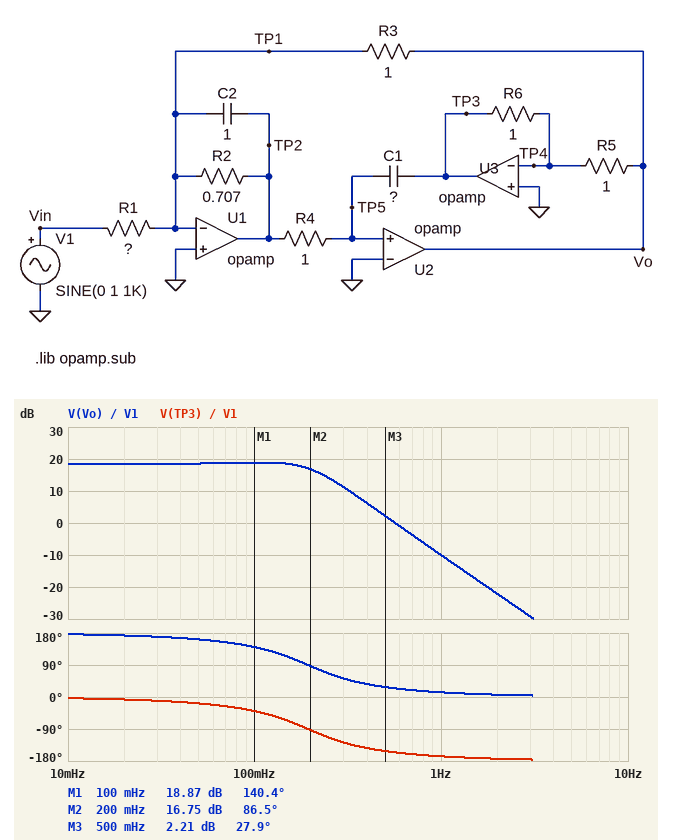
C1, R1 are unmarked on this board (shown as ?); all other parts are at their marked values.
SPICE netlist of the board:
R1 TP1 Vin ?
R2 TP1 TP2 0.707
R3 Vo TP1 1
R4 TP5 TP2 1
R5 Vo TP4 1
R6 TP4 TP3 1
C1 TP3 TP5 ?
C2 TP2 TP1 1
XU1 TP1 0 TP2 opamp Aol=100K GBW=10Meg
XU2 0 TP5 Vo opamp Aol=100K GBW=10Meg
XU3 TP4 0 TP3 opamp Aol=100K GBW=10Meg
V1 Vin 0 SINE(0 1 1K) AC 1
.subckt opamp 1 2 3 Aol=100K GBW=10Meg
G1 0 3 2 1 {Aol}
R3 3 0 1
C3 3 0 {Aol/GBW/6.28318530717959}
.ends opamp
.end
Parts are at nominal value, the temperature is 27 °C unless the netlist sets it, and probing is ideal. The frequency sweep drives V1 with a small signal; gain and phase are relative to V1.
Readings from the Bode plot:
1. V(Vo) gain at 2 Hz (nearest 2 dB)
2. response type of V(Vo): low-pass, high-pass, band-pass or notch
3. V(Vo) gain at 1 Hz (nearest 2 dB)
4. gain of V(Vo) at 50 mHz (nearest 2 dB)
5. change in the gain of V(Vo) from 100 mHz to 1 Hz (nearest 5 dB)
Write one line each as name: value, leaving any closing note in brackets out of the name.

V(Vo) gain at 2 Hz: -22 dB
response type of V(Vo): low-pass, high-pass, band-pass or notch: low-pass
V(Vo) gain at 1 Hz: -10 dB
gain of V(Vo) at 50 mHz: 18 dB
change in the gain of V(Vo) from 100 mHz to 1 Hz: -30 dB
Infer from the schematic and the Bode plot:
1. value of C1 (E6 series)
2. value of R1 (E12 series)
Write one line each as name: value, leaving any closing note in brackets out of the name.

value of C1: 680 mF
value of R1: 0.12 Ω
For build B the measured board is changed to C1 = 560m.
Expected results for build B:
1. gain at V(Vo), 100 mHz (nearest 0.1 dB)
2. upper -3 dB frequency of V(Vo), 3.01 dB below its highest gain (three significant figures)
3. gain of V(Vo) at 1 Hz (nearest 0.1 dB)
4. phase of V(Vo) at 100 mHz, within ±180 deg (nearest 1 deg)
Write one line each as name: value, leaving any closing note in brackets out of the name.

gain at V(Vo), 100 mHz: 19.1 dB
upper -3 dB frequency of V(Vo), 3.01 dB below its highest gain: 246 mHz
gain of V(Vo) at 1 Hz: -8.3 dB
phase of V(Vo) at 100 mHz, within ±180 deg: 147 deg
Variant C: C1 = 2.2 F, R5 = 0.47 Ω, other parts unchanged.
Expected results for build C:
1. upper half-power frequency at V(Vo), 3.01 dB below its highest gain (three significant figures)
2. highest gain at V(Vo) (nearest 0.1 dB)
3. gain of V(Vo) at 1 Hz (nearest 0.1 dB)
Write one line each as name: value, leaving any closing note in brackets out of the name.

upper half-power frequency at V(Vo), 3.01 dB below its highest gain: 26.9 mHz
highest gain at V(Vo): 18.4 dB
gain of V(Vo) at 1 Hz: -27.1 dB
